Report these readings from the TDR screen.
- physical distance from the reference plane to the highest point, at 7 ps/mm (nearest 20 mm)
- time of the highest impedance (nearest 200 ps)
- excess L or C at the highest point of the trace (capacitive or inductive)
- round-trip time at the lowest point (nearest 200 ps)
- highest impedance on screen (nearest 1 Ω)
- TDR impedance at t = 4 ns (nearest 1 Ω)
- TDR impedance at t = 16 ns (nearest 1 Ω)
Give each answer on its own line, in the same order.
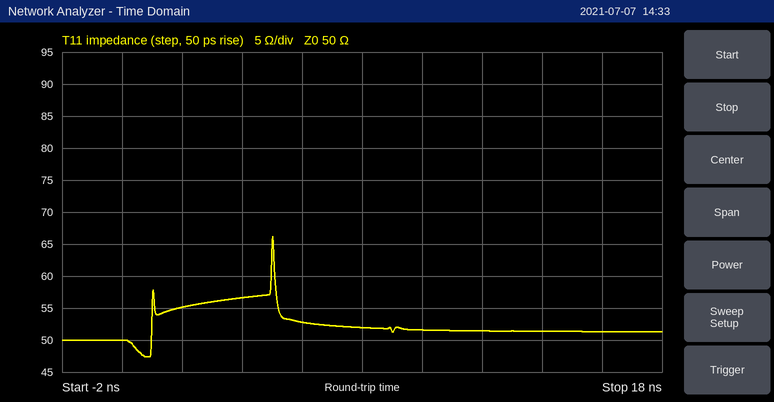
360 mm
5.0 ns
inductive
800 ps
66 Ω
57 Ω
51 Ω
